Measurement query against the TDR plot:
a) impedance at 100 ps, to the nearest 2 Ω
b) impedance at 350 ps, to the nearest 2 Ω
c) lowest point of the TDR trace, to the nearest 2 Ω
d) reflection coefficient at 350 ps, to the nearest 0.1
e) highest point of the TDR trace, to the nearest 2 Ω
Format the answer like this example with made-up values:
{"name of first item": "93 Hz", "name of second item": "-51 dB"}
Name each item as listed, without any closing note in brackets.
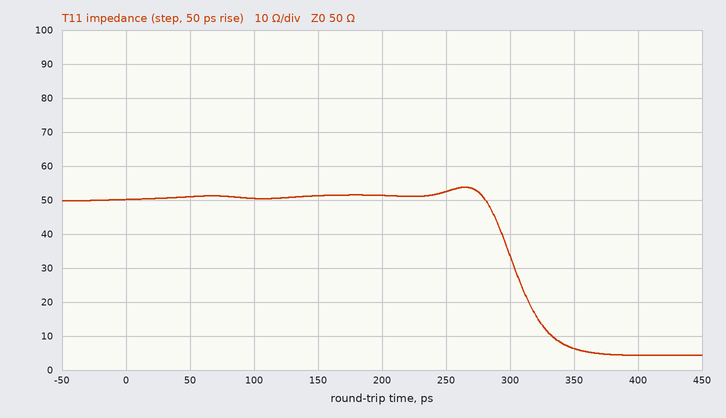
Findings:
{"impedance at 100 ps, to the nearest 2 Ω": "50 Ω", "impedance at 350 ps, to the nearest 2 Ω": "6 Ω", "lowest point of the TDR trace, to the nearest 2 Ω": "4 Ω", "reflection coefficient at 350 ps, to the nearest 0.1": "-0.8", "highest point of the TDR trace, to the nearest 2 Ω": "54 Ω"}
